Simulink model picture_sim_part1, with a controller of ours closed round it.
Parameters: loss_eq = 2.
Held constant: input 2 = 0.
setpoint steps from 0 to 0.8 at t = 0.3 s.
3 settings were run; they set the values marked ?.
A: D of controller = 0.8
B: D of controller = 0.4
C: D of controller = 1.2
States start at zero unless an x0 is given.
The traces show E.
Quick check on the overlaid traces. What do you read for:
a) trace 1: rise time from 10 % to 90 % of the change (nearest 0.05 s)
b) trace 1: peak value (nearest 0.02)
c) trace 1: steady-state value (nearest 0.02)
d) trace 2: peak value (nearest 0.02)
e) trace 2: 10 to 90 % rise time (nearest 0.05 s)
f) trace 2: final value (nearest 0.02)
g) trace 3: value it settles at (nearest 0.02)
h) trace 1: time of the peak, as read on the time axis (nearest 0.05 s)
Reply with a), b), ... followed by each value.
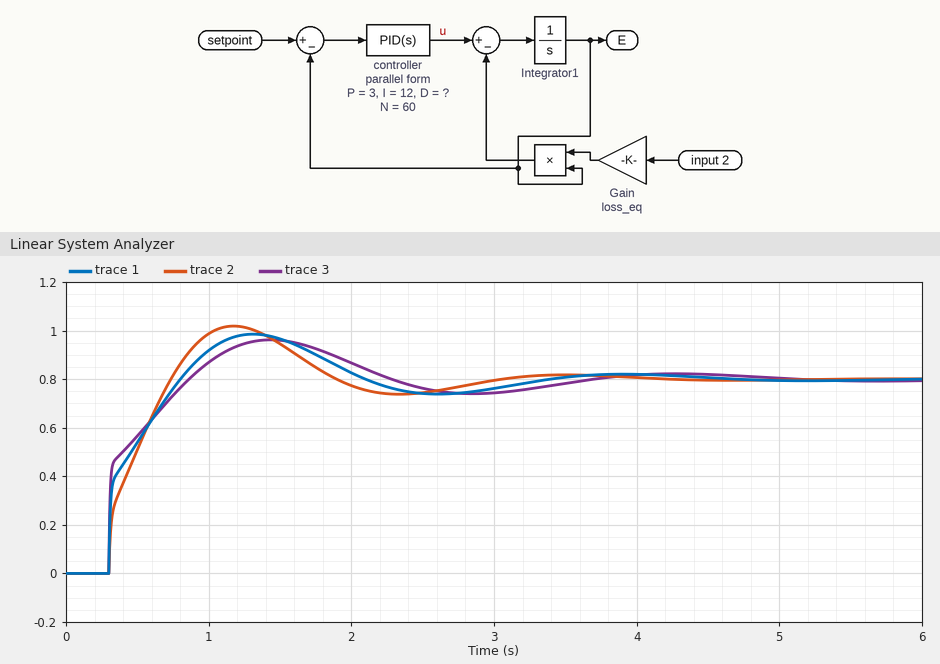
a) 0.40 s
b) 0.98
c) 0.80
d) 1.02
e) 0.35 s
f) 0.80
g) 0.80
h) 1.30 s
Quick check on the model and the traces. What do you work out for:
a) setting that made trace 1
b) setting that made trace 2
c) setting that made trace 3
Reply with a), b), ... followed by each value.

a) A
b) B
c) C
